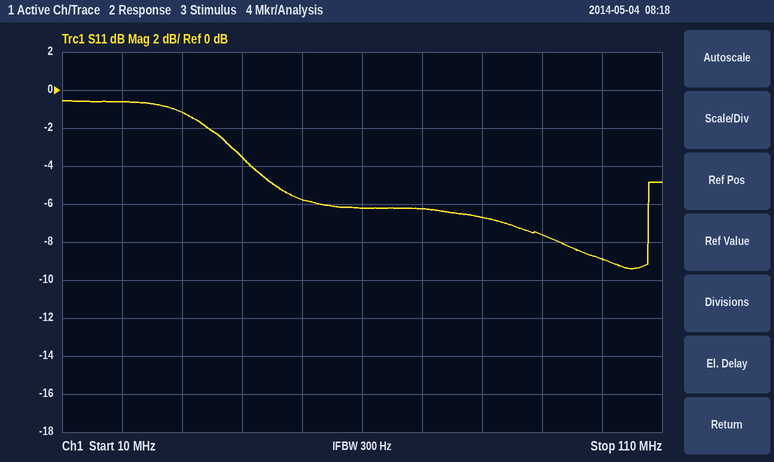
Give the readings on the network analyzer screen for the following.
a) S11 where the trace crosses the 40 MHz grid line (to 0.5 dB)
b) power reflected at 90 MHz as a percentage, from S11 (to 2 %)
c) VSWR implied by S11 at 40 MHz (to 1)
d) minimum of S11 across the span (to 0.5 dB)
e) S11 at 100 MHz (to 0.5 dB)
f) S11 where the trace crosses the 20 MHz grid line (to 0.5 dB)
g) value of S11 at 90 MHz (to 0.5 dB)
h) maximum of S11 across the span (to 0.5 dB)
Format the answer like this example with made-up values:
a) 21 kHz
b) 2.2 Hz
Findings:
a) -3.5 dB
b) 18 %
c) 5
d) -9.5 dB
e) -9.0 dB
f) -0.5 dB
g) -7.5 dB
h) -0.5 dB
